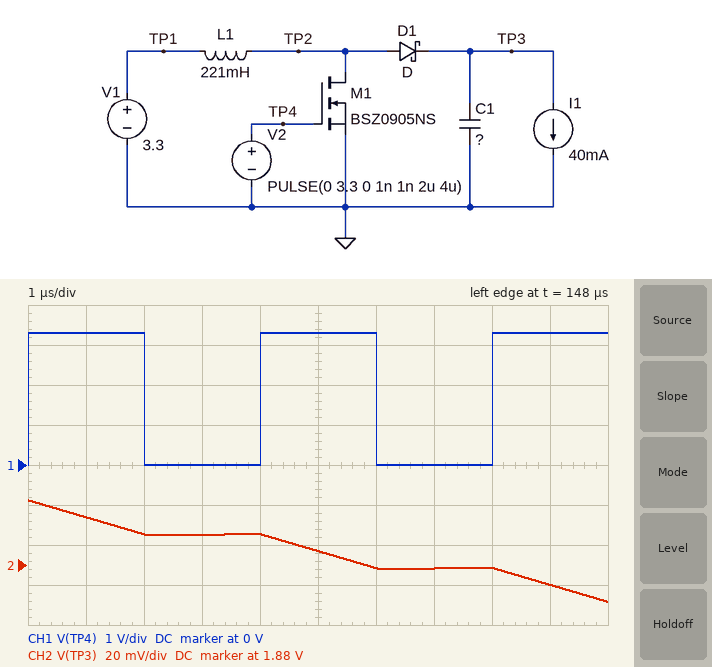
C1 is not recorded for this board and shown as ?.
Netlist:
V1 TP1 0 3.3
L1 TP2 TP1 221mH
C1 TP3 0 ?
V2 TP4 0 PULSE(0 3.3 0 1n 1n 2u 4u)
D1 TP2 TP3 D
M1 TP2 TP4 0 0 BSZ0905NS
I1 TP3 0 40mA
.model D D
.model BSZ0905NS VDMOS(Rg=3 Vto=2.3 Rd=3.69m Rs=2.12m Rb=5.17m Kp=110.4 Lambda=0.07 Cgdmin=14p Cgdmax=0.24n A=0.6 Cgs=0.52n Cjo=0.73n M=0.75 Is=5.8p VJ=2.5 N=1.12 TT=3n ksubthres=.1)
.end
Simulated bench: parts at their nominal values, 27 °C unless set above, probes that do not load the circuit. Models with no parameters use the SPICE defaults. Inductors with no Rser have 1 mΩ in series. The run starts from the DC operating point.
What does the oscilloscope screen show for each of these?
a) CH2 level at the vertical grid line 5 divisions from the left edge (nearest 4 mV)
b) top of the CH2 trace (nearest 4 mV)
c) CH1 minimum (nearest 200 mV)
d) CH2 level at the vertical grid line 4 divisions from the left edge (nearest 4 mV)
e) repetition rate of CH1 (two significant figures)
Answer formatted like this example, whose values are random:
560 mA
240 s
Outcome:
1.888 V
1.912 V
0 V
1.896 V
250 kHz
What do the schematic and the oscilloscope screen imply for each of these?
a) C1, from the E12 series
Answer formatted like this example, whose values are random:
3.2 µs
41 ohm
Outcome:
4.7 µF
